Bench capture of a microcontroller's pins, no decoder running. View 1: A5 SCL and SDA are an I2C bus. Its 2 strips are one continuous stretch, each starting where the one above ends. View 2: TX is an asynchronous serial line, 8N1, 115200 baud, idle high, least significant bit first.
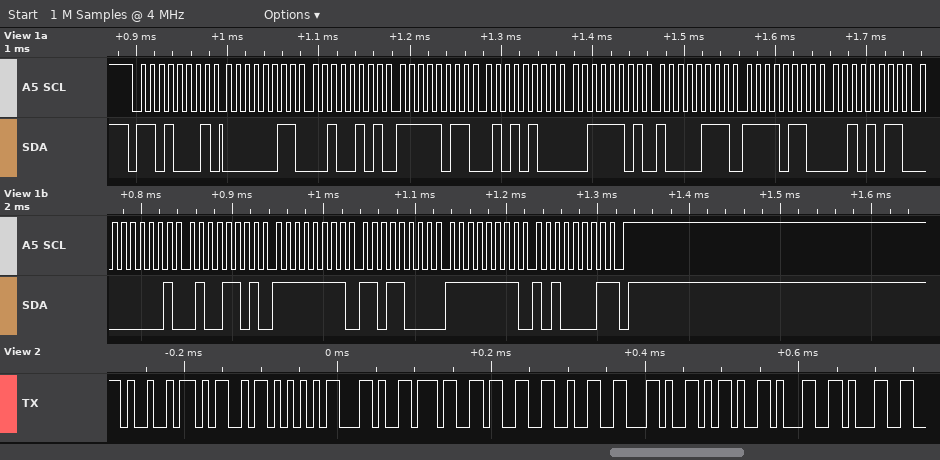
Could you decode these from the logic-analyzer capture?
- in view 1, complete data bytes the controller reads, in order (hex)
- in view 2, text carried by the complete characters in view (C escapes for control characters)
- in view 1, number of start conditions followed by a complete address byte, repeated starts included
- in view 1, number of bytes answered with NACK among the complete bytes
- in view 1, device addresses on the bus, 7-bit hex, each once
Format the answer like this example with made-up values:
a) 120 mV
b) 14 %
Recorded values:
a) 03 25 FB 54 3D 87 F6 2B 01 4D FF D8 FF A1
b) "IMU,732,-11"
c) 1
d) 1
e) 0x68
